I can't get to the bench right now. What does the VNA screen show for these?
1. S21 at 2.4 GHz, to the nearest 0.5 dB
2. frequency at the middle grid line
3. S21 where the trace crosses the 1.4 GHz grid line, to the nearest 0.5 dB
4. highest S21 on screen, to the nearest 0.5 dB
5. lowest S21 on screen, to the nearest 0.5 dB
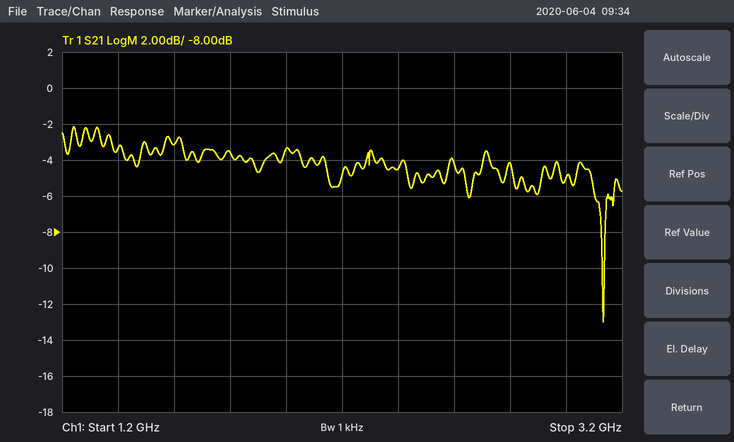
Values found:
-4.5 dB
2.2 GHz
-3.5 dB
-2.0 dB
-13.0 dB
